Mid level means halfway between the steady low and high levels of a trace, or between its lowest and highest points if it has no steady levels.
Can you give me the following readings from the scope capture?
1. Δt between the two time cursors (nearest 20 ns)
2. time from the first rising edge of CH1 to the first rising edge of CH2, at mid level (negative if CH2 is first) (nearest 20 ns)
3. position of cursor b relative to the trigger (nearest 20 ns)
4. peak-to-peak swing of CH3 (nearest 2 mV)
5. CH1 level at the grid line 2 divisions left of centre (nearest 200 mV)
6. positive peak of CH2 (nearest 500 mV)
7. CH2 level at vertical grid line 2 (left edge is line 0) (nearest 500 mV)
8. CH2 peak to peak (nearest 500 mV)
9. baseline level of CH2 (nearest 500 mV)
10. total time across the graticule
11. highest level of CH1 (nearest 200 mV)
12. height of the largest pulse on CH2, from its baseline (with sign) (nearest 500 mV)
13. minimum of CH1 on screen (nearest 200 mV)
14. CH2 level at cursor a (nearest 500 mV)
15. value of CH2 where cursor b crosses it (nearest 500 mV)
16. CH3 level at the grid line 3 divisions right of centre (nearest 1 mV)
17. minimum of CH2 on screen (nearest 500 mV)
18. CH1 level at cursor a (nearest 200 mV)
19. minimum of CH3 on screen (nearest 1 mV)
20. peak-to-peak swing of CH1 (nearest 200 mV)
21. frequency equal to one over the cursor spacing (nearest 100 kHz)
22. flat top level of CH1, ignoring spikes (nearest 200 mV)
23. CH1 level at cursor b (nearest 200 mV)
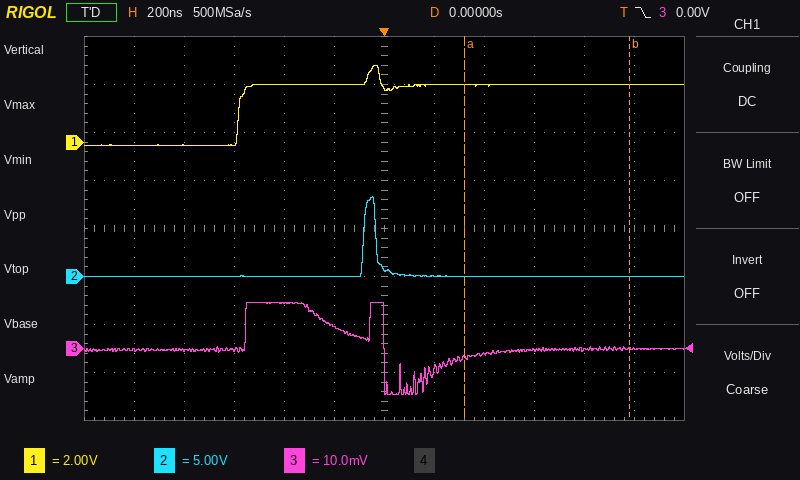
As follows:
660 ns
+500 ns
+980 ns
20 mV
2.4 V
8.5 V
0.0 V
8.5 V
0.0 V
2.4 µs
3.2 V
+8.5 V
-200 mV
0.0 V
0.0 V
0 mV
0.0 V
2.4 V
-10 mV
3.4 V
1.5 MHz
2.4 V
2.4 V
